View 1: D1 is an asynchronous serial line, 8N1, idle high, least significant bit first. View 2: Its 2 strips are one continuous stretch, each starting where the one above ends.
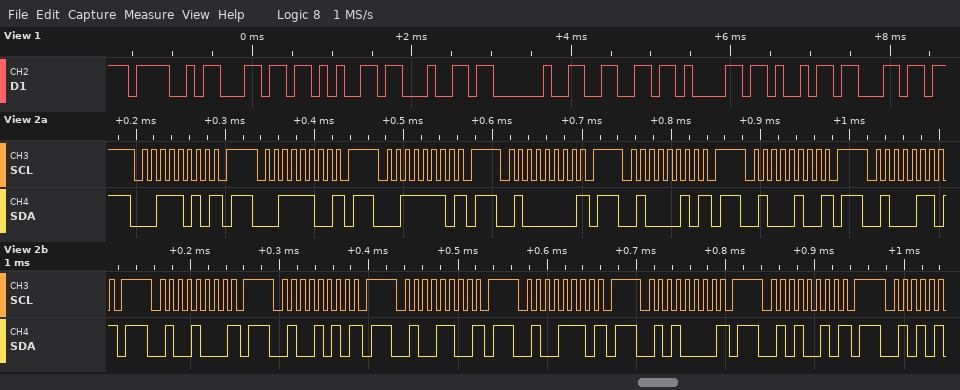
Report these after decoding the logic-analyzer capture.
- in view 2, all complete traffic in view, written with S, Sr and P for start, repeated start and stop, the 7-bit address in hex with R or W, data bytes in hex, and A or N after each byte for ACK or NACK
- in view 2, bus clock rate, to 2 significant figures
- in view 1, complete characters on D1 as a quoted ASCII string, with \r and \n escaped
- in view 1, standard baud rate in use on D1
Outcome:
S 1DW N P S 1EW N P S 1FW N P S 20W N P S 21W N P S 22W N P S 23W N P S 24W N P S 25W N P S 26W N P S 27W N P S 28W N P S 29W N P
100 kHz
"Oled fail"
9600 baud
